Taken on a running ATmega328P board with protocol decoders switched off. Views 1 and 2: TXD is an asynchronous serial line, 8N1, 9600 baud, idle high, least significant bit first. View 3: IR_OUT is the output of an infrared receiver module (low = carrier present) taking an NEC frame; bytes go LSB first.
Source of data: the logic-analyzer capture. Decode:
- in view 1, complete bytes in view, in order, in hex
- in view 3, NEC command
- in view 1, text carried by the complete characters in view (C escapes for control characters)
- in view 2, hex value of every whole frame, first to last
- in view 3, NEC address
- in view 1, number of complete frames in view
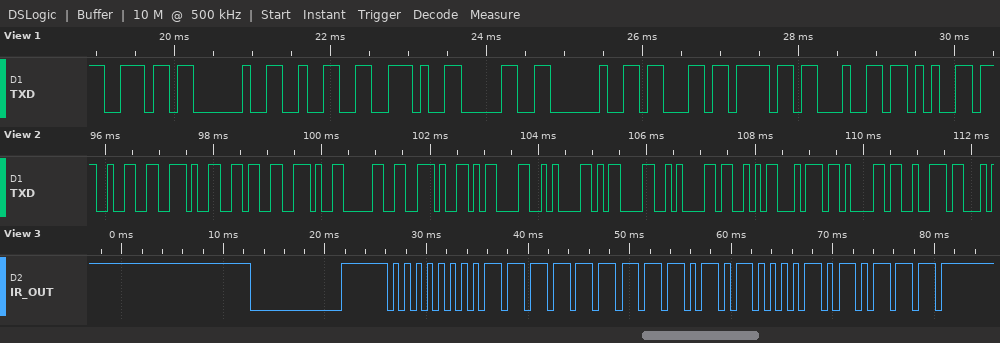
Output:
6E 20 32 2E 30 20 63 6F 64 65
0x15
"n 2.0 code"
32 2E 36 2E 30 2E 0D 0A 0D 0A 53 74 61 72
0x00
10
